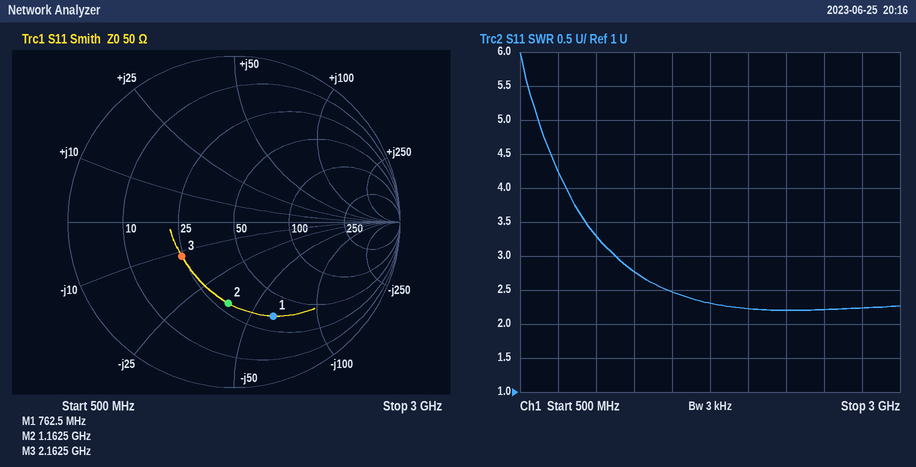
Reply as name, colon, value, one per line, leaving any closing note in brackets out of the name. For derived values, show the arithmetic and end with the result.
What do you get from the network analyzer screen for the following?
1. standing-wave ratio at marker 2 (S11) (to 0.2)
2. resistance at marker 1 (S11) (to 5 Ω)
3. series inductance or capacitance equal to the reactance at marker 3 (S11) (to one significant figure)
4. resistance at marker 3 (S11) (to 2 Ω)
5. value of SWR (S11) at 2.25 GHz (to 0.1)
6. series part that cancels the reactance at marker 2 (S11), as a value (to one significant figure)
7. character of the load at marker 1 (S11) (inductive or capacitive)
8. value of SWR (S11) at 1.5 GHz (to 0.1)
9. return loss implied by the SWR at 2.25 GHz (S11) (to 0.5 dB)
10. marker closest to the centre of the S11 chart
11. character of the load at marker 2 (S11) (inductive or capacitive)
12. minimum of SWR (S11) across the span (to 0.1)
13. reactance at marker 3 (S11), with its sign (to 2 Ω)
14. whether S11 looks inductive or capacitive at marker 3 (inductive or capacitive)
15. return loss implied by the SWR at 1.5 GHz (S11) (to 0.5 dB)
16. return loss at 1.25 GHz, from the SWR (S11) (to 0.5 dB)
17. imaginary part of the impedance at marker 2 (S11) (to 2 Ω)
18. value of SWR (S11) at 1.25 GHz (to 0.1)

standing-wave ratio at marker 2 (S11): 3.0
resistance at marker 1 (S11): 35 Ω
series inductance or capacitance equal to the reactance at marker 3 (S11): C = 1/(2π × 2.1625 GHz × 12 Ω) ≈ 6 pF
resistance at marker 3 (S11): 24 Ω
value of SWR (S11) at 2.25 GHz: 2.2
series part that cancels the reactance at marker 2 (S11), as a value: L = 38 Ω/(2π × 1.1625 GHz) ≈ 5 nH
character of the load at marker 1 (S11): capacitive
value of SWR (S11) at 1.5 GHz: 2.5
return loss implied by the SWR at 2.25 GHz (S11): −20 log10((2.2 − 1)/(2.2 + 1)) ≈ 8.5 dB
marker closest to the centre of the S11 chart: marker 3
character of the load at marker 2 (S11): capacitive
minimum of SWR (S11) across the span: 2.2
reactance at marker 3 (S11), with its sign: -12 Ω
whether S11 looks inductive or capacitive at marker 3: capacitive
return loss implied by the SWR at 1.5 GHz (S11): −20 log10((2.5 − 1)/(2.5 + 1)) ≈ 7.36 dB, so 7.5 dB to the nearest 0.5 dB
return loss at 1.25 GHz, from the SWR (S11): −20 log10((2.8 − 1)/(2.8 + 1)) ≈ 6.5 dB
imaginary part of the impedance at marker 2 (S11): -38 Ω
value of SWR (S11) at 1.25 GHz: 2.8
